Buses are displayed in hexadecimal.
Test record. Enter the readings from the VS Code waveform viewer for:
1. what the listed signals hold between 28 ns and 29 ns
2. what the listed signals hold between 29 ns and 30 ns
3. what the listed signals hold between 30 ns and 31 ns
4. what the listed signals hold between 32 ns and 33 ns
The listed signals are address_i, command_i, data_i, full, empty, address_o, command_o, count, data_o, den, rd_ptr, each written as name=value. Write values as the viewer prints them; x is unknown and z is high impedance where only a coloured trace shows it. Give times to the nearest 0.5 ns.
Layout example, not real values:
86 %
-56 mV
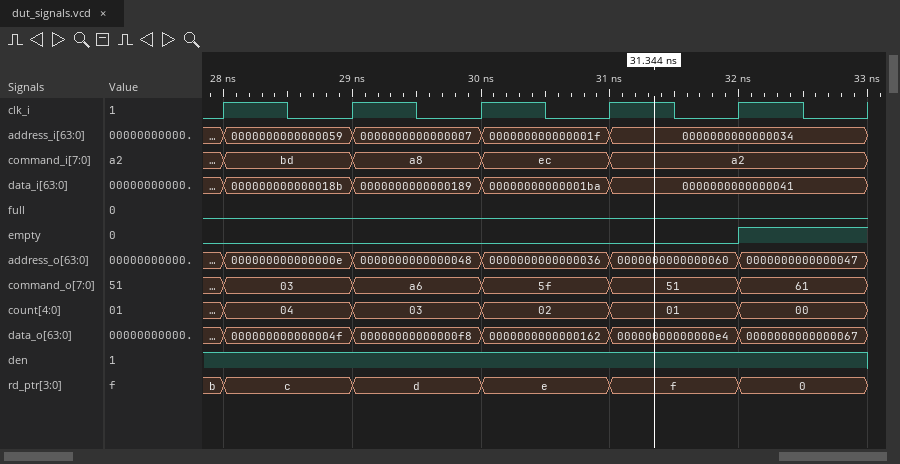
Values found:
address_i=0000000000000059, command_i=bd, data_i=000000000000018b, full=0, empty=0, address_o=000000000000000e, command_o=03, count=04, data_o=000000000000004f, den=1, rd_ptr=c
address_i=0000000000000007, command_i=a8, data_i=0000000000000189, full=0, empty=0, address_o=0000000000000048, command_o=a6, count=03, data_o=00000000000000f8, den=1, rd_ptr=d
address_i=000000000000001f, command_i=ec, data_i=00000000000001ba, full=0, empty=0, address_o=0000000000000036, command_o=5f, count=02, data_o=0000000000000162, den=1, rd_ptr=e
address_i=0000000000000034, command_i=a2, data_i=0000000000000041, full=0, empty=1, address_o=0000000000000047, command_o=61, count=00, data_o=0000000000000067, den=1, rd_ptr=0
